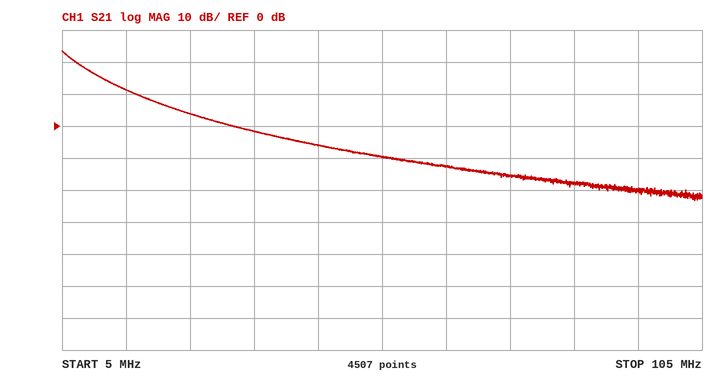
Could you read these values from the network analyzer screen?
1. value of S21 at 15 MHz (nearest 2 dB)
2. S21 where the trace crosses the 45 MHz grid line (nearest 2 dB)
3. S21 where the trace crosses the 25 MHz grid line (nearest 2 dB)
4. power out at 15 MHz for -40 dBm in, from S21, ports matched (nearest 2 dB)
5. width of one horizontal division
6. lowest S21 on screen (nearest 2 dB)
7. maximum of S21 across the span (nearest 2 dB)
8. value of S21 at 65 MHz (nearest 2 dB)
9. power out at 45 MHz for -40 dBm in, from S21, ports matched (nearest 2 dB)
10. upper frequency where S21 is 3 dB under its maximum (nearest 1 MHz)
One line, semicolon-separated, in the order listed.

12 dB; -6 dB; 4 dB; -28 dBm; 10 MHz; -24 dB; 24 dB; -12 dB; -46 dBm; 7 MHz
